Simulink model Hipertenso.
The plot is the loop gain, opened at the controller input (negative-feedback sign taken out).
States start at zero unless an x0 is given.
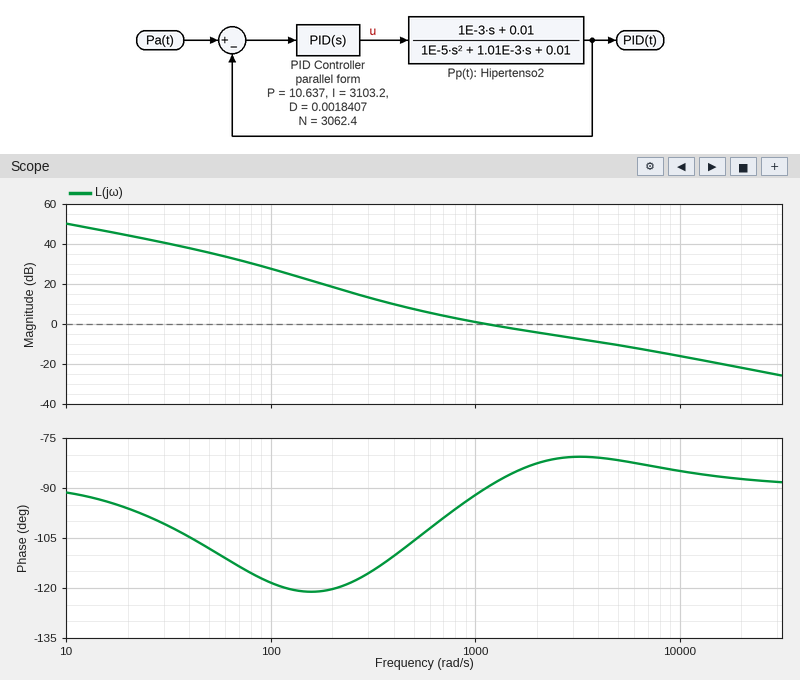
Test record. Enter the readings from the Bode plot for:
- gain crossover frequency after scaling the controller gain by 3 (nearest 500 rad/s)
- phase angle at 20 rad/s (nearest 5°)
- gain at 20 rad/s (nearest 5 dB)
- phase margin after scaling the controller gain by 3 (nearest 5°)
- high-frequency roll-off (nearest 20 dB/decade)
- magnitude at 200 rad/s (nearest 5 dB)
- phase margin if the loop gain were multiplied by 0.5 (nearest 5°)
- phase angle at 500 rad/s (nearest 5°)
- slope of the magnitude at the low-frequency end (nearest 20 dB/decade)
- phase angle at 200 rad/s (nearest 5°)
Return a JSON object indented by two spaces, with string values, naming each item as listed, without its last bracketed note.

{
  "gain crossover frequency after scaling the controller gain by 3": "4500 rad/s",
  "phase angle at 20 rad/s": "-95°",
  "gain at 20 rad/s": "45 dB",
  "phase margin after scaling the controller gain by 3": "100°",
  "high-frequency roll-off": "-20 dB/decade",
  "magnitude at 200 rad/s": "20 dB",
  "phase margin if the loop gain were multiplied by 0.5": "75°",
  "phase angle at 500 rad/s": "-105°",
  "slope of the magnitude at the low-frequency end": "-20 dB/decade",
  "phase angle at 200 rad/s": "-120°"
}
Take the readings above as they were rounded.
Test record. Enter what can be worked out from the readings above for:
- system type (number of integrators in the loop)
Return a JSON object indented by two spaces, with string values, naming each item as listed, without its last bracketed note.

{
  "system type": "1"
}
